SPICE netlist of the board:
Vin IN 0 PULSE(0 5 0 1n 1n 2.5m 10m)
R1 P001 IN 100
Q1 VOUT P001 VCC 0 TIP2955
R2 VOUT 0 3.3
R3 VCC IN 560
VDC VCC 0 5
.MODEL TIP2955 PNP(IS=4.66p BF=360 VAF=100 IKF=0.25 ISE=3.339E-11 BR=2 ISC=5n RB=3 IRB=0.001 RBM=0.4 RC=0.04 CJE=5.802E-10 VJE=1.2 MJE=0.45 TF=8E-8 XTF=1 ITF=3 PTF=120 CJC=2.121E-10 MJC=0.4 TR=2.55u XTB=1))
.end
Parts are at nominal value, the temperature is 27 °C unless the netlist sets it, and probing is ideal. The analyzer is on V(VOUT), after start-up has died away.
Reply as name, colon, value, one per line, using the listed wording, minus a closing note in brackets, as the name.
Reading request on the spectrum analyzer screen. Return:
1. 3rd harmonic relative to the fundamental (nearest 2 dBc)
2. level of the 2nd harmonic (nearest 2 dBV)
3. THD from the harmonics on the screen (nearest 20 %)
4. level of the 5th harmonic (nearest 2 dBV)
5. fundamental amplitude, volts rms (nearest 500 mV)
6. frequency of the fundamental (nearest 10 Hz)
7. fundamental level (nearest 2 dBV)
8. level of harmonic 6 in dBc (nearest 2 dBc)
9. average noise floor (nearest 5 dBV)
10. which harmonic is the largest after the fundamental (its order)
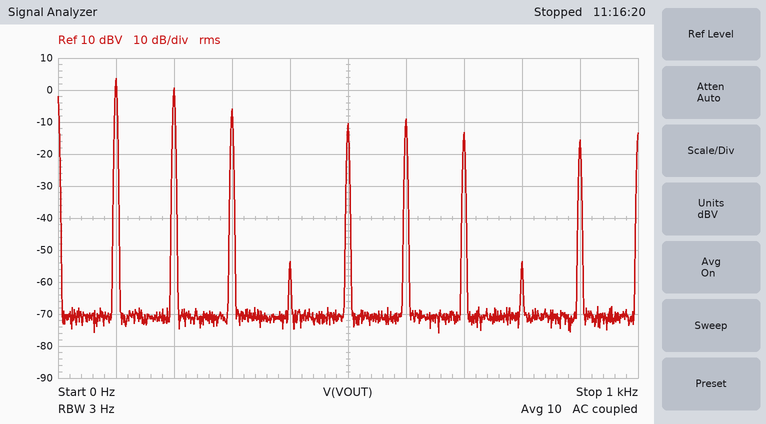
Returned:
3rd harmonic relative to the fundamental: -10 dBc
level of the 2nd harmonic: 0 dBV
THD from the harmonics on the screen: 80 %
level of the 5th harmonic: -10 dBV
fundamental amplitude, volts rms: 1.5 V
frequency of the fundamental: 100 Hz
fundamental level: 4 dBV
level of harmonic 6 in dBc: -12 dBc
average noise floor: -70 dBV
which harmonic is the largest after the fundamental: 2
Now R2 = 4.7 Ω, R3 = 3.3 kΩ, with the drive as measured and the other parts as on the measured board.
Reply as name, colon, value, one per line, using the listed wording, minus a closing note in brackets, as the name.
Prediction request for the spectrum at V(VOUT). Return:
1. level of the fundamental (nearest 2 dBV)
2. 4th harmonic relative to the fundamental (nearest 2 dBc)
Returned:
level of the fundamental: 4 dBV
4th harmonic relative to the fundamental: -52 dBc
